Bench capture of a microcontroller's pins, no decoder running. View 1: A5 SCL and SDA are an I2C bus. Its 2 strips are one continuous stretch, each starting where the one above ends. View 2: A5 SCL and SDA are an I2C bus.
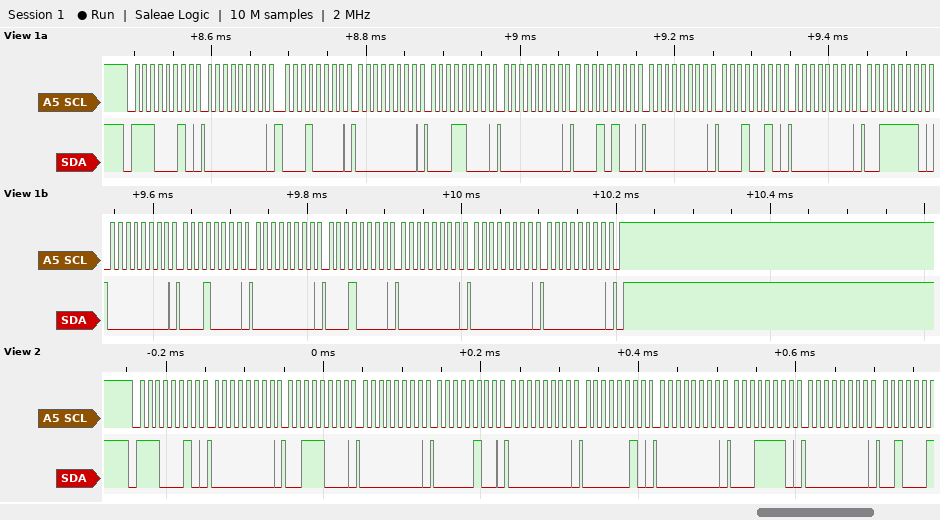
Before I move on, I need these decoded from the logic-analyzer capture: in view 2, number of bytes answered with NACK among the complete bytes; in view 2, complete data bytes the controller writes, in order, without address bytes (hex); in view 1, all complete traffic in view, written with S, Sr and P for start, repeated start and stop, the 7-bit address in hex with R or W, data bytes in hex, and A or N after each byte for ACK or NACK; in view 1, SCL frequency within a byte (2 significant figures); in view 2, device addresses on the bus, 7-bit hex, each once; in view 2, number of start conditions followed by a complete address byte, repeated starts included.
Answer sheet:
0
00 38 00 04 00 02 00 1E 00
S 71W A 00 A 10 A 00 A 18 A 00 A 14 A 00 A 12 A 00 A 3E A 00 A 10 A 00 A 10 A 00 A 00 A 00 A P
100 kHz
0x71
1
